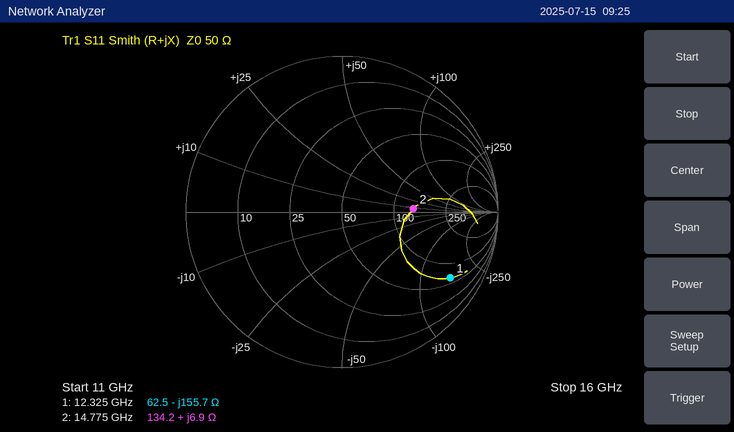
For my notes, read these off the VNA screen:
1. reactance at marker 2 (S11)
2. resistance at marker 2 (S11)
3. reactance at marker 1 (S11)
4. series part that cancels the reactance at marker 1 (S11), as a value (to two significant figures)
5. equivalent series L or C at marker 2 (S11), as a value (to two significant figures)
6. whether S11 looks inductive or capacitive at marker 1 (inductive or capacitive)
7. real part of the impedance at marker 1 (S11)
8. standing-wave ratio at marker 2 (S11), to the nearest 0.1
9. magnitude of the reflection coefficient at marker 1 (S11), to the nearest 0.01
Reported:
+6.9 Ω
134.2 Ω
-155.7 Ω
2.0 nH
74 pH
capacitive
62.5 Ω
2.7
0.81
